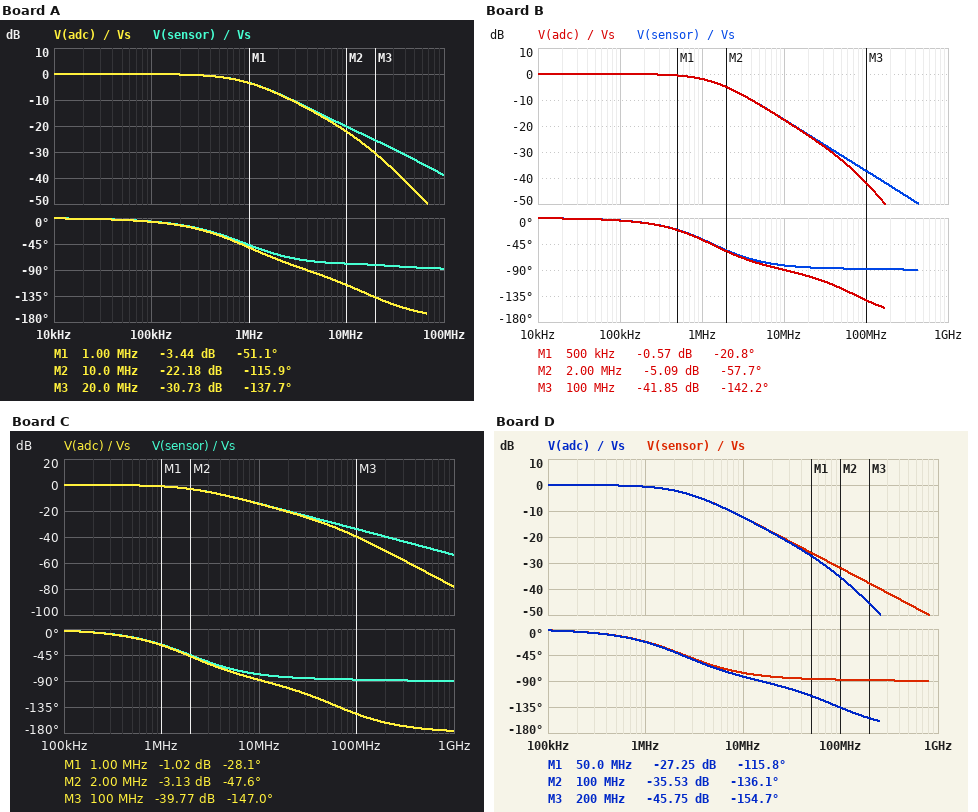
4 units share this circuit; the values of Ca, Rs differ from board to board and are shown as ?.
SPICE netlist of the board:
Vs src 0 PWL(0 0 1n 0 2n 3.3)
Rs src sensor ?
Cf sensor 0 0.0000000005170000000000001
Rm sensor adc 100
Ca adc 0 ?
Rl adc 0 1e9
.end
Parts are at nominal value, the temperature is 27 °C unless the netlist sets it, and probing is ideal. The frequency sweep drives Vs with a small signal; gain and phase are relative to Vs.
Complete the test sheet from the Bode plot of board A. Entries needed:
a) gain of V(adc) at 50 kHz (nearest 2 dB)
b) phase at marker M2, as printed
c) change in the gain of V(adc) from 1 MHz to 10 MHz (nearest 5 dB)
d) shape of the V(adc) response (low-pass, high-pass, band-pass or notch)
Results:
0 dB
-115.9 deg
-20 dB
low-pass
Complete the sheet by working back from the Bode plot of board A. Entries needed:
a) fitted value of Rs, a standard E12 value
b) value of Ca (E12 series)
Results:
270 Ω
120 pF
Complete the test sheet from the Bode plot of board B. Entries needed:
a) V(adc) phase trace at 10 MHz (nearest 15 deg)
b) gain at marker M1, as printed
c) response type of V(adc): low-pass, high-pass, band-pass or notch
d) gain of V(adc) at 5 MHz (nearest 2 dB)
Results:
-90 deg
-0.57 dB
low-pass
-12 dB
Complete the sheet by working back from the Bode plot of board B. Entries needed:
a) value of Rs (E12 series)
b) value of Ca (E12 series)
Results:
220 Ω
22 pF
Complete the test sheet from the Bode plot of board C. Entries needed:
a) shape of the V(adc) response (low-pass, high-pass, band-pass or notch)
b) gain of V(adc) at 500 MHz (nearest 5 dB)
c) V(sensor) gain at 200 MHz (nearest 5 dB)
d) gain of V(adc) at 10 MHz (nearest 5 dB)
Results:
low-pass
-65 dB
-40 dB
-15 dB
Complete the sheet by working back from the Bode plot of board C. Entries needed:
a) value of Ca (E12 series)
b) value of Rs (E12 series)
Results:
27 pF
150 Ω
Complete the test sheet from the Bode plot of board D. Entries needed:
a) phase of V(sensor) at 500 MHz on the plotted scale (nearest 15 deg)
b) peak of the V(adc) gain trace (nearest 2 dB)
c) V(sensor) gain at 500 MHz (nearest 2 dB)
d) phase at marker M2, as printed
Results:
-90 deg
0 dB
-46 dB
-136.1 deg
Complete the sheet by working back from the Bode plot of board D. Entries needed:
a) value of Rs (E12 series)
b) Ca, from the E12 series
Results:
120 Ω
18 pF
